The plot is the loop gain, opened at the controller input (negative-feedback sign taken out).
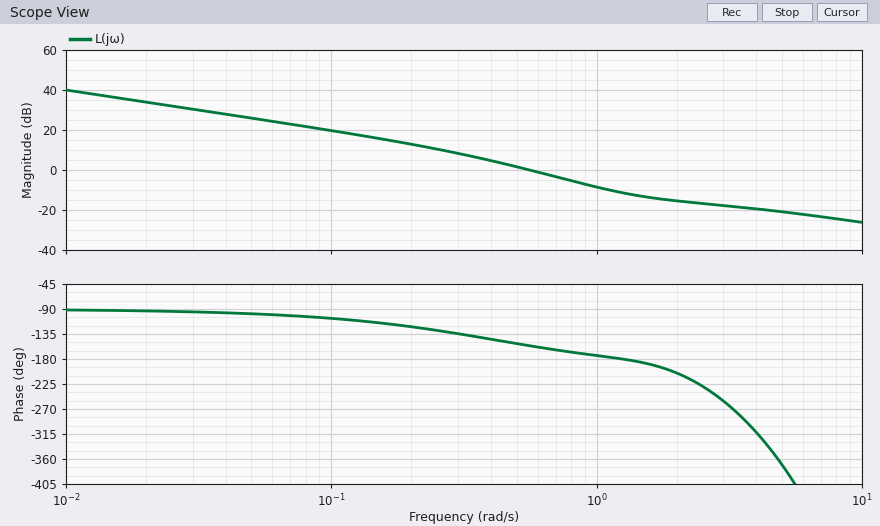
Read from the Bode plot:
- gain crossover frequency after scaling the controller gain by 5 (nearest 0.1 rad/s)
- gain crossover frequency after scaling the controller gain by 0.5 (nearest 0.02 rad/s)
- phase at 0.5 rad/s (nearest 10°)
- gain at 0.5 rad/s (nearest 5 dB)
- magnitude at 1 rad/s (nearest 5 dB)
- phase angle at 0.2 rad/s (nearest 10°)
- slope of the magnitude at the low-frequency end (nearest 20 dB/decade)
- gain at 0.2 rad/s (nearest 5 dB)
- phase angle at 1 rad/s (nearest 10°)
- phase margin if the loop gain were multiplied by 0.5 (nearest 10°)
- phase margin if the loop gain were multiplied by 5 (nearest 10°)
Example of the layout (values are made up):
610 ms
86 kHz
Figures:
1.6 rad/s
0.36 rad/s
-150°
0 dB
-10 dB
-120°
-20 dB/decade
15 dB
-170°
40°
-10°
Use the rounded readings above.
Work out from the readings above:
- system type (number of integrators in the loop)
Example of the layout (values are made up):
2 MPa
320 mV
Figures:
1
